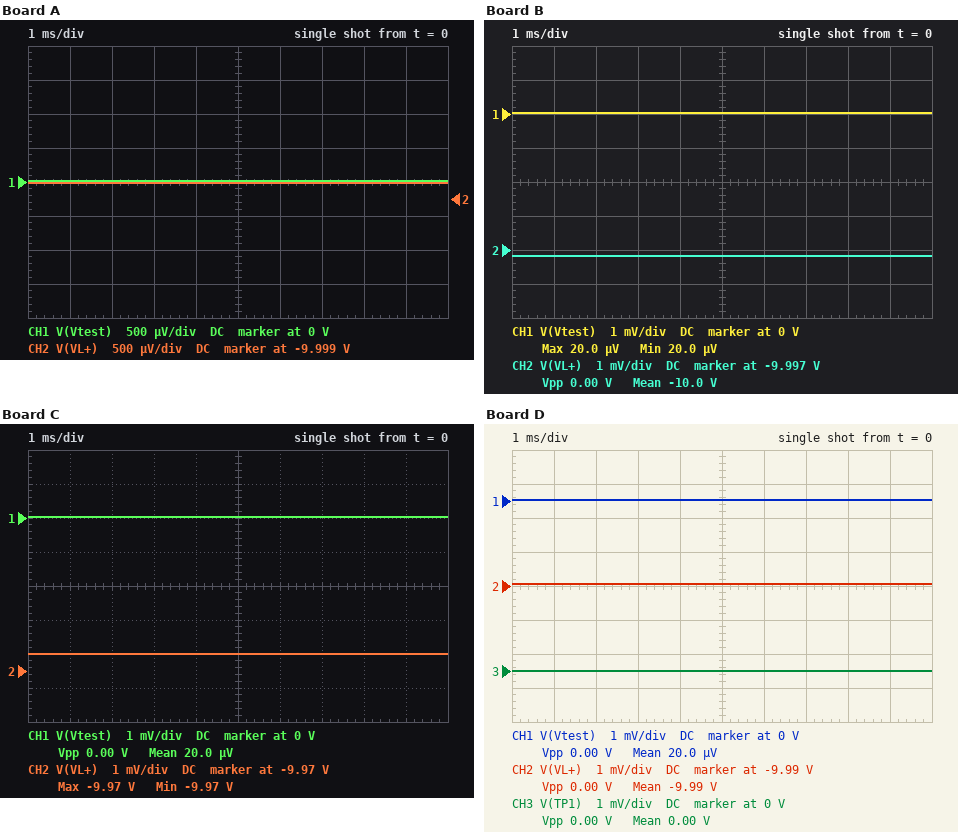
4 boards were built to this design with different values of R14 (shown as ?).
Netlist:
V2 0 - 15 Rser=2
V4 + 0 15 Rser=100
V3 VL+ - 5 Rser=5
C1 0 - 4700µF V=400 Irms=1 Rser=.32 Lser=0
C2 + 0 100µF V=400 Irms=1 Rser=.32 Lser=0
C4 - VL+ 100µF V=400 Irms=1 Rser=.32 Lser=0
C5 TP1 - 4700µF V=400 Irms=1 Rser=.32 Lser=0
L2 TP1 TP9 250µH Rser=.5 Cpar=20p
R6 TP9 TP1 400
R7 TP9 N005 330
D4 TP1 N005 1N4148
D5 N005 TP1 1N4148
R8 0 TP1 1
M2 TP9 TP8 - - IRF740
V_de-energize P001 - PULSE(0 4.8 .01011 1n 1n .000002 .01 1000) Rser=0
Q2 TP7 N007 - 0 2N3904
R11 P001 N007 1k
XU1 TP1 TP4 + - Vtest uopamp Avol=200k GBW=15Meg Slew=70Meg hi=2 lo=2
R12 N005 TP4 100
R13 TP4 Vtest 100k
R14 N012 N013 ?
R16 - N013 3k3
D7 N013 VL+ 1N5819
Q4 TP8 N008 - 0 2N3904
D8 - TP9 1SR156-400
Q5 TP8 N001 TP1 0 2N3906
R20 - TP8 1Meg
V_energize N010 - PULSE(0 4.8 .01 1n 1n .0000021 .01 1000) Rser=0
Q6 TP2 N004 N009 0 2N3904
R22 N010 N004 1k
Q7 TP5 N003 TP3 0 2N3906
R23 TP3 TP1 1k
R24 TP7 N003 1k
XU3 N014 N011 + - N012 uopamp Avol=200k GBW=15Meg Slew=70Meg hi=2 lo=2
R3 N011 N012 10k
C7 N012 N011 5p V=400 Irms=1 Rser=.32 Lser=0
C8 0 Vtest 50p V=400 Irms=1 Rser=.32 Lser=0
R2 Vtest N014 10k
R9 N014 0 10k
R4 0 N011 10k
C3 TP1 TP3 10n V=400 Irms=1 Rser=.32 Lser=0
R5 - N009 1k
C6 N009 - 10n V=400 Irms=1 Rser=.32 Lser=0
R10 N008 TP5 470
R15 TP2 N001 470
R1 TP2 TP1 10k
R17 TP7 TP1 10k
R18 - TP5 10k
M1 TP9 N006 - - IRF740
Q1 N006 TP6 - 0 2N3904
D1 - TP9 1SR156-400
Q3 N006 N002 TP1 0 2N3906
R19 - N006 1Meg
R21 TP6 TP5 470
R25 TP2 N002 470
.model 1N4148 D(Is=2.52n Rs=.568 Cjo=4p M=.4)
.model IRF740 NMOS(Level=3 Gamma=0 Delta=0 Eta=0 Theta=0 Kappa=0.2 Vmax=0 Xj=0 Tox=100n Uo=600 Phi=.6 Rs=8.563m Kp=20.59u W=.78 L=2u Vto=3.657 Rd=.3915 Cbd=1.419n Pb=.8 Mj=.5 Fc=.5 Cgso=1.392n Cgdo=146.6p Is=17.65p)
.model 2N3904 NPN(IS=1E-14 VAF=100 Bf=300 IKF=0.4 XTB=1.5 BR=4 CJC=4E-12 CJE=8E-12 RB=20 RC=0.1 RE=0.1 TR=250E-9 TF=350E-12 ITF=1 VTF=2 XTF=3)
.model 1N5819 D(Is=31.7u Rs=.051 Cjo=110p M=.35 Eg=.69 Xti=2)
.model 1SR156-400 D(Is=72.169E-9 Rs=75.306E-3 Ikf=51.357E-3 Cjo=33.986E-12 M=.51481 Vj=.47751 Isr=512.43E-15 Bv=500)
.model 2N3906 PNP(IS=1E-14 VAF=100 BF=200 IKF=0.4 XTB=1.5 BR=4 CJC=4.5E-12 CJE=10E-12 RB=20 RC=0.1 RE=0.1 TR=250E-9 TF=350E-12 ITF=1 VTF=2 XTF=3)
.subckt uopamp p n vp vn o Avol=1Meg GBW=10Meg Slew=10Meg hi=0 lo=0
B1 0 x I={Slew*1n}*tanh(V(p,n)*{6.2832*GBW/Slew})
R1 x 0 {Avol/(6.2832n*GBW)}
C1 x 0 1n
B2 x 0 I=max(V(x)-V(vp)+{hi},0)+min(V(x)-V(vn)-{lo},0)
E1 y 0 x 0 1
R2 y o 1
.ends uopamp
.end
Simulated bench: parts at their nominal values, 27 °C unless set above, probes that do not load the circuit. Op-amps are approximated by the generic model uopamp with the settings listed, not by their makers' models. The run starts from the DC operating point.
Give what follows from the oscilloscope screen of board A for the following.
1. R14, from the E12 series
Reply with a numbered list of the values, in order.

1. 18 kΩ
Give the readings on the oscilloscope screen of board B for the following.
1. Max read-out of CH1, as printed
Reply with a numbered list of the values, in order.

1. 20.0 µV
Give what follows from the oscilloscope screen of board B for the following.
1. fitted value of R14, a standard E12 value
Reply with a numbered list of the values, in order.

1. 6.8 kΩ
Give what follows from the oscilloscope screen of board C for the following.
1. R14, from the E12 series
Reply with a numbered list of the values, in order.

1. 1.8 kΩ
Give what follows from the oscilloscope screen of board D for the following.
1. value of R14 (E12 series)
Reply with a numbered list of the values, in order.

1. 3.9 kΩ
